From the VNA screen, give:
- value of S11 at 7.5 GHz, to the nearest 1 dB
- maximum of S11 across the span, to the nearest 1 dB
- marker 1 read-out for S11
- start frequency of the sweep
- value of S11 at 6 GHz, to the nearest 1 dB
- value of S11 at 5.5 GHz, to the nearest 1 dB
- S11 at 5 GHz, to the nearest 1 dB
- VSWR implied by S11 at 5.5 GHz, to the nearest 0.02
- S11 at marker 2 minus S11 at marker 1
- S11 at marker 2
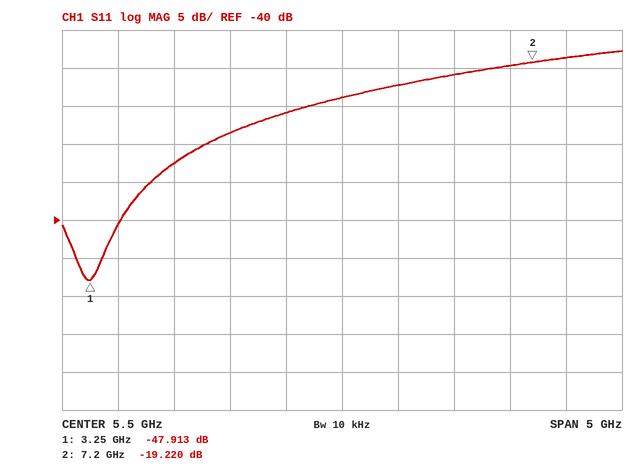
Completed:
-19 dB
-18 dB
-47.913 dB
3 GHz
-22 dB
-24 dB
-26 dB
1.14
28.693 dB
-19.220 dB
